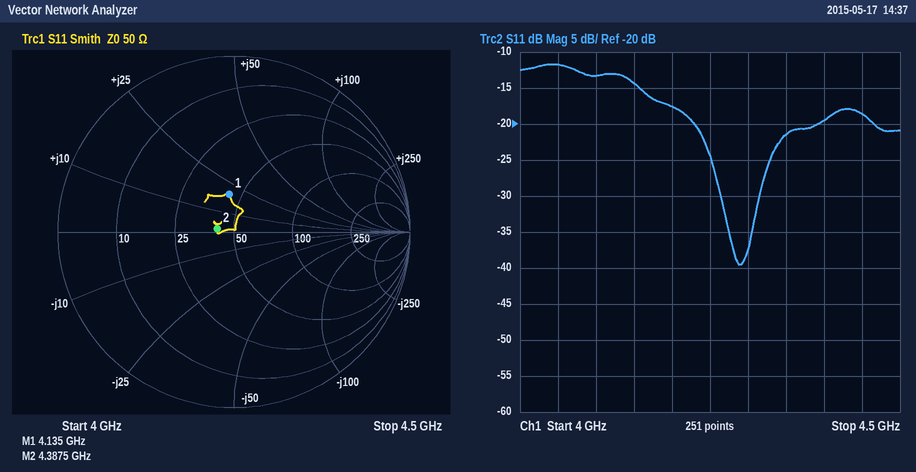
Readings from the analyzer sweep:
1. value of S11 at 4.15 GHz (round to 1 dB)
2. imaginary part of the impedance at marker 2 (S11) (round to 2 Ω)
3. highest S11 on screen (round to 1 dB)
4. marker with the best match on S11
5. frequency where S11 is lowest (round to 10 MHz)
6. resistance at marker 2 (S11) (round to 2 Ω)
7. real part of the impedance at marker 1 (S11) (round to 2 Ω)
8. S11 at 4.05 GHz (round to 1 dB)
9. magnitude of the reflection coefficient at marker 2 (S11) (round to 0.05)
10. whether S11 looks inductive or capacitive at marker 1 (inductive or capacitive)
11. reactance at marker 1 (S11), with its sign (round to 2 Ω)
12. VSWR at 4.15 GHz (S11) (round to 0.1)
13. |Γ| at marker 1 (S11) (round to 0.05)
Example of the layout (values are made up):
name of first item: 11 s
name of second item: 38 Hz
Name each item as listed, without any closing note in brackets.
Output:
value of S11 at 4.15 GHz: -14 dB
imaginary part of the impedance at marker 2 (S11): +2 Ω
highest S11 on screen: -12 dB
marker with the best match on S11: marker 2
frequency where S11 is lowest: 4.29 GHz
resistance at marker 2 (S11): 42 Ω
real part of the impedance at marker 1 (S11): 44 Ω
S11 at 4.05 GHz: -12 dB
magnitude of the reflection coefficient at marker 2 (S11): 0.10
whether S11 looks inductive or capacitive at marker 1: inductive
reactance at marker 1 (S11), with its sign: +20 Ω
VSWR at 4.15 GHz (S11): 1.5
|Γ| at marker 1 (S11): 0.20
